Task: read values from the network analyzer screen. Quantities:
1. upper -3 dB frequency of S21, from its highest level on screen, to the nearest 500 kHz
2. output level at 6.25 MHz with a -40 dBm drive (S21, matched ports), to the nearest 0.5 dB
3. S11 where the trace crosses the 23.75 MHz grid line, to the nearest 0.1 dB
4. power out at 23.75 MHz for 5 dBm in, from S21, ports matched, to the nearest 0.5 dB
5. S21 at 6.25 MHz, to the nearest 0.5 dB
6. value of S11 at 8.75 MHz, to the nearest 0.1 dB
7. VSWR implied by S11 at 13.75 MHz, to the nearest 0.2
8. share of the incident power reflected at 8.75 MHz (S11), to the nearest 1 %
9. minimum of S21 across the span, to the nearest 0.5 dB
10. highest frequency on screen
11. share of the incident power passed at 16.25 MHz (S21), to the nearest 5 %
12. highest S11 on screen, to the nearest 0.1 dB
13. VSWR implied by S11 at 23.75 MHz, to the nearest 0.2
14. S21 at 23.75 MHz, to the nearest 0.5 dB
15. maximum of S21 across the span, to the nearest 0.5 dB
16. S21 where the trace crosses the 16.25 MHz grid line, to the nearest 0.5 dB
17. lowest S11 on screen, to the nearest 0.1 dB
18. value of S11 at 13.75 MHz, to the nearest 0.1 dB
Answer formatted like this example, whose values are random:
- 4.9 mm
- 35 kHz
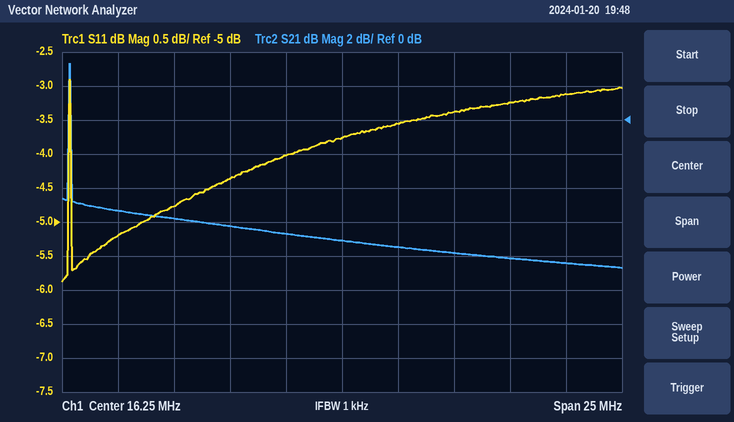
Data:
- 4.0 MHz
- -45.5 dBm
- -3.2 dB
- -3.0 dBm
- -5.5 dB
- -4.8 dB
- 4.4
- 33 %
- -8.5 dB
- 28.75 MHz
- 20 %
- -2.9 dB
- 5.4
- -8.0 dB
- 3.5 dB
- -7.0 dB
- -5.9 dB
- -4.0 dB
